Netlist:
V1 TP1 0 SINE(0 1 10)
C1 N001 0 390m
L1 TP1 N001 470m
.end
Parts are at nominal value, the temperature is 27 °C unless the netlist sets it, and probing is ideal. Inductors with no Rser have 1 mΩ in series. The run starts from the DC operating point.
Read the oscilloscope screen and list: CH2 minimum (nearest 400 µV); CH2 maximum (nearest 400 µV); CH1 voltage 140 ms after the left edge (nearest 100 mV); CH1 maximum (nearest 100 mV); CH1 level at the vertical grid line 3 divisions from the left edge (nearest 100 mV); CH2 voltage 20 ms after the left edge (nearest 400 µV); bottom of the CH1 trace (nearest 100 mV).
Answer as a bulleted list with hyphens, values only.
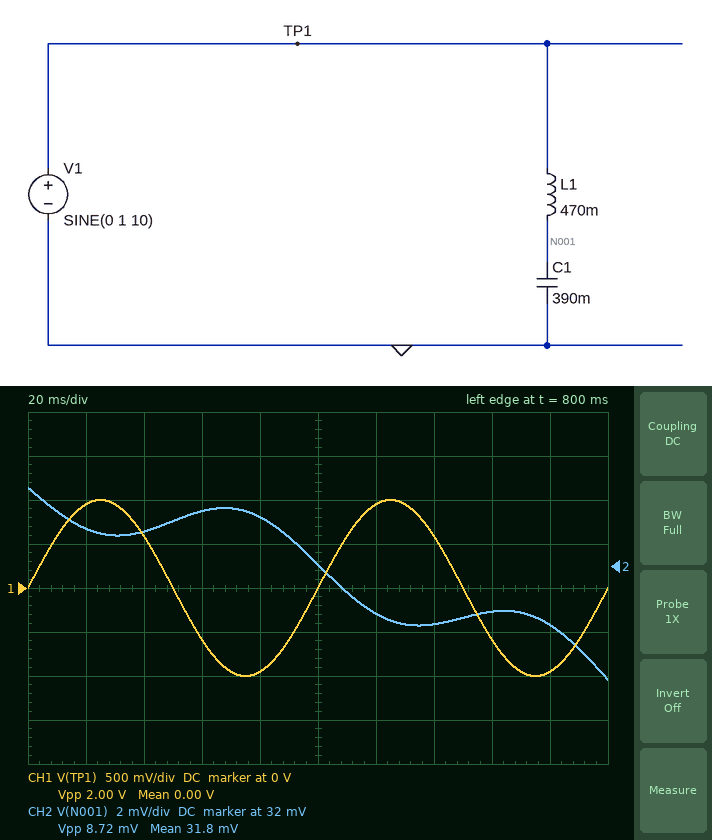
- 26.8 mV
- 35.6 mV
- 600 mV
- 1.0 V
- -600 mV
- 33.6 mV
- -1.0 V
